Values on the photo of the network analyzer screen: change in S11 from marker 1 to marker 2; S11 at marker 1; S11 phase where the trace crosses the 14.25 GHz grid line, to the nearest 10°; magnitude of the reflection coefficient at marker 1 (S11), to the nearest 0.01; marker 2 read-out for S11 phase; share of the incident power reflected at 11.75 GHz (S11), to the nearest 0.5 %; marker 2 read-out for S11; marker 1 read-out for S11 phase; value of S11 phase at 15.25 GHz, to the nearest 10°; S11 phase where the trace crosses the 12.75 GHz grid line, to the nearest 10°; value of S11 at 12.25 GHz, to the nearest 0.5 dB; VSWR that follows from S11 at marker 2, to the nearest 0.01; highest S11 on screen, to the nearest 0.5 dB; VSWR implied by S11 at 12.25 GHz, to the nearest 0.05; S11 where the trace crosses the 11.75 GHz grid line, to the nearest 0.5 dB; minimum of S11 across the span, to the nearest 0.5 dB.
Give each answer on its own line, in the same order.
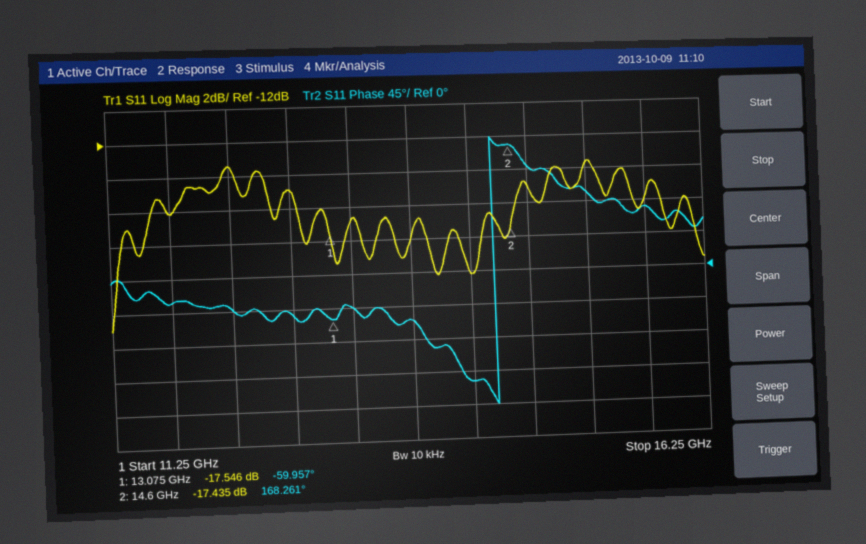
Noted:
0.111 dB
-17.546 dB
-150°
0.13
168.261°
2.5 %
-17.435 dB
-59.957°
100°
-50°
-13.5 dB
1.31
-13.5 dB
1.55
-16.0 dB
-23.0 dB
